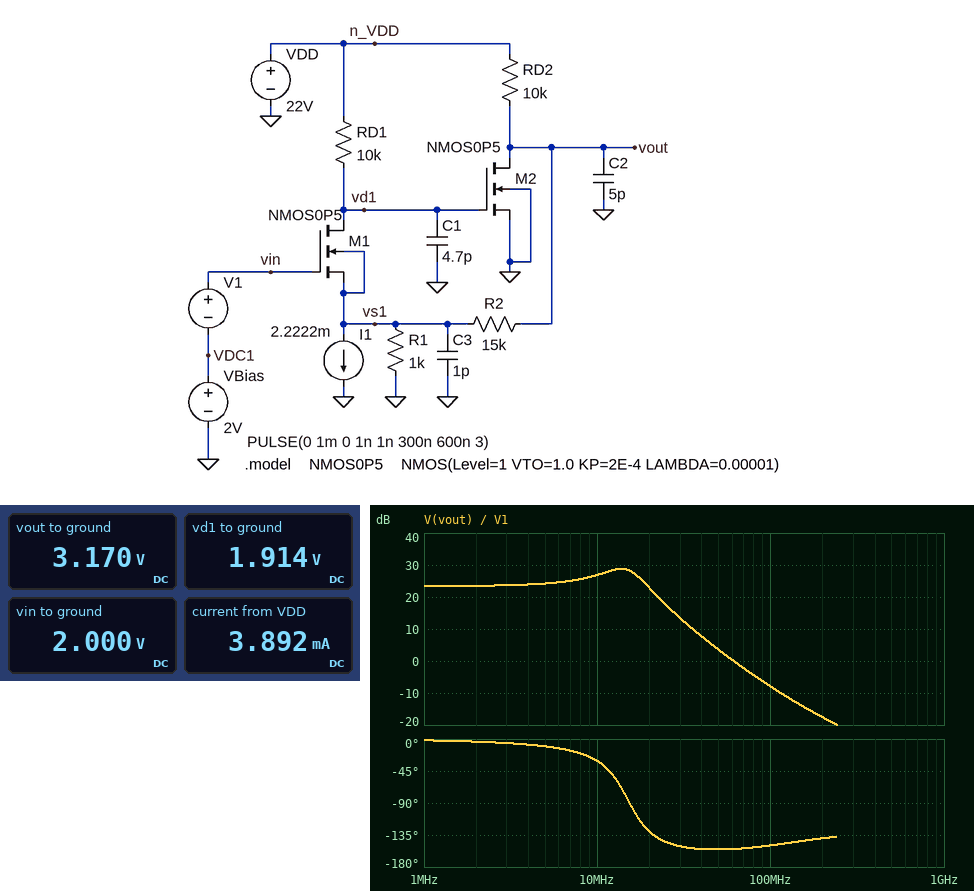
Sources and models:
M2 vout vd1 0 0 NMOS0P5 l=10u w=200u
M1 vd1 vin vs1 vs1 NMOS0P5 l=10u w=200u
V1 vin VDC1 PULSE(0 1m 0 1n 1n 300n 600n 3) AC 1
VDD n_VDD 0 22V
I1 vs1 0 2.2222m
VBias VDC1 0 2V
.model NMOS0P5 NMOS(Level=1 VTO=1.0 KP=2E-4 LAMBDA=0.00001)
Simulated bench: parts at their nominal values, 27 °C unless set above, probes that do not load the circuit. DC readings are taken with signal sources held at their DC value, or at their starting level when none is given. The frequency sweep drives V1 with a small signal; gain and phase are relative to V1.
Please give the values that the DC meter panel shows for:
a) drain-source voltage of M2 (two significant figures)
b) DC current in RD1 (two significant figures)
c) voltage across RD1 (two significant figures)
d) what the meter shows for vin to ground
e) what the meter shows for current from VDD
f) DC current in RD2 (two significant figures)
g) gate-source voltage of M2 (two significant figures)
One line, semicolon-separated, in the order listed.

3.2 V; 2.0 mA; 20 V; 2.000 V; 3.892 mA; 1.9 mA; 1.9 V
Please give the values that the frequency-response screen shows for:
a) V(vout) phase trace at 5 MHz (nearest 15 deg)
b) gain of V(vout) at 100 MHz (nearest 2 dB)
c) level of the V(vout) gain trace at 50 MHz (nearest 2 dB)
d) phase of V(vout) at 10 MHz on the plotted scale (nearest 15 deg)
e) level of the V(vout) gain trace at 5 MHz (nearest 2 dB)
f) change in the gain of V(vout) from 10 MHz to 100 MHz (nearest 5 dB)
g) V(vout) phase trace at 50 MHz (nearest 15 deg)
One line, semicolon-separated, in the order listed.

-15 deg; -8 dB; 4 dB; -30 deg; 24 dB; -35 dB; -150 deg
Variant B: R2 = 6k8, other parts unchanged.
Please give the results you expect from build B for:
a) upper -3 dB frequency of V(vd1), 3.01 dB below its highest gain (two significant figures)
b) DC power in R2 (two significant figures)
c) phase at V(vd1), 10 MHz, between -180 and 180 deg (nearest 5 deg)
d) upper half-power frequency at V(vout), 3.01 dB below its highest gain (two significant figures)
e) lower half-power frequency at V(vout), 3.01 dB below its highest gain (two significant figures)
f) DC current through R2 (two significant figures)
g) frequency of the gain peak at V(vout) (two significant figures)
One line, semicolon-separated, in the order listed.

28 MHz; 320 µW; -140 deg; 26 MHz; 15 MHz; 220 µA; 21 MHz
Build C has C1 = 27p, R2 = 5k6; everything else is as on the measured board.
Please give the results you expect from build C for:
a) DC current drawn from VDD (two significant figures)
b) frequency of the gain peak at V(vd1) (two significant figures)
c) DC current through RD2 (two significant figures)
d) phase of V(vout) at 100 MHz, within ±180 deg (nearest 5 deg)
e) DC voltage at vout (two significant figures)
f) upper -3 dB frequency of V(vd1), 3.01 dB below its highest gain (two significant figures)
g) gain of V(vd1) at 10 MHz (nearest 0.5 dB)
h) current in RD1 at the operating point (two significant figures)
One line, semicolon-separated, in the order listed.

4.1 mA; 9.4 MHz; 2.1 mA; -130 deg; 1.2 V; 14 MHz; -2.5 dB; 2.0 mA
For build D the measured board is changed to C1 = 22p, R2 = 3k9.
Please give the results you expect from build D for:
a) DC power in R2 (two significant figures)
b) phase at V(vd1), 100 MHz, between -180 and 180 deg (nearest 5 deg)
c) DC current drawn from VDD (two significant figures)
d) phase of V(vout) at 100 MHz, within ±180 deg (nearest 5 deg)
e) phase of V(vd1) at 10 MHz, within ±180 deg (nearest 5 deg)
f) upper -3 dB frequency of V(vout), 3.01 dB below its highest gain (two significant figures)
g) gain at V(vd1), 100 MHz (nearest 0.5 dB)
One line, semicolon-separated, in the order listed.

190 µW; 110 deg; 4.1 mA; -120 deg; 130 deg; 8.1 MHz; -22.0 dB
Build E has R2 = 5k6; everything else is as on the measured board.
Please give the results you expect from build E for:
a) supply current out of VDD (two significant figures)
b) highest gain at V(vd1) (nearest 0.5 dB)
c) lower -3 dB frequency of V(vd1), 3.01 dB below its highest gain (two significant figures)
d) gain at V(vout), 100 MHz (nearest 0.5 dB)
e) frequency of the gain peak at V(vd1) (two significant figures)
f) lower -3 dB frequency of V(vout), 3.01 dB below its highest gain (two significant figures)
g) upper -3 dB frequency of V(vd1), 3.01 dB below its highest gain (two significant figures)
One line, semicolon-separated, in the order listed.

4.1 mA; 9.0 dB; 19 MHz; -6.5 dB; 24 MHz; 16 MHz; 31 MHz
